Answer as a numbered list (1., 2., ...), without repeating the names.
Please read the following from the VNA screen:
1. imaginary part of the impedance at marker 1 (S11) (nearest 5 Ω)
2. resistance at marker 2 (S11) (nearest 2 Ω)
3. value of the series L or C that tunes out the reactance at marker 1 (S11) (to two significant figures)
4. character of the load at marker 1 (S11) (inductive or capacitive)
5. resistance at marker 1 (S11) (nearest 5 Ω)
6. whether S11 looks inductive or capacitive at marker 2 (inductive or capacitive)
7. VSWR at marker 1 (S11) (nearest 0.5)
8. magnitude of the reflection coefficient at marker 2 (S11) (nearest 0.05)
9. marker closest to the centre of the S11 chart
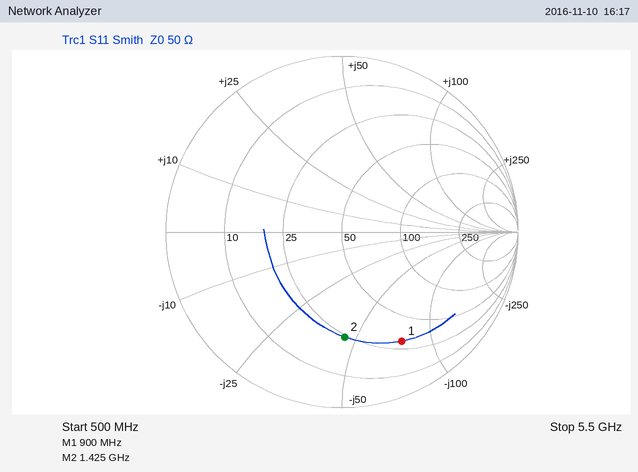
1. -75 Ω
2. 24 Ω
3. 13 nH
4. capacitive
5. 30 Ω
6. capacitive
7. 6.0
8. 0.60
9. marker 2
